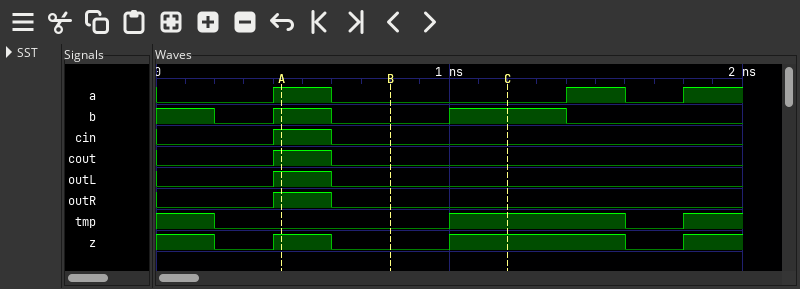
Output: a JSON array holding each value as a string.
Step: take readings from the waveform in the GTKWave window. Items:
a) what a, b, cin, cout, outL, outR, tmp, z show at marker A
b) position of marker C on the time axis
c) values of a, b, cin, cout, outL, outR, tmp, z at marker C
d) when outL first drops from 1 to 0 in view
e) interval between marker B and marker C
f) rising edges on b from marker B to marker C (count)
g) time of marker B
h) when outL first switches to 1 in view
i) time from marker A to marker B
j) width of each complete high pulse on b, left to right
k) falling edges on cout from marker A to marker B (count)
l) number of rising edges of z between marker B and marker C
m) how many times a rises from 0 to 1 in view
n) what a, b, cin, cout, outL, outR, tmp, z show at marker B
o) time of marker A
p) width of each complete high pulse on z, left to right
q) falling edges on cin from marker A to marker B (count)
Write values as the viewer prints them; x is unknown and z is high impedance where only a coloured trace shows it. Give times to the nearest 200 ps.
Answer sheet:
["a=1, b=1, cin=1, cout=1, outL=1, outR=1, tmp=0, z=1", "1200 ps", "a=0, b=1, cin=0, cout=0, outL=0, outR=0, tmp=1, z=1", "600 ps", "400 ps", "1", "800 ps", "400 ps", "400 ps", "200 ps, 400 ps", "1", "1", "3", "a=0, b=0, cin=0, cout=0, outL=0, outR=0, tmp=0, z=0", "400 ps", "200 ps, 600 ps", "1"]
